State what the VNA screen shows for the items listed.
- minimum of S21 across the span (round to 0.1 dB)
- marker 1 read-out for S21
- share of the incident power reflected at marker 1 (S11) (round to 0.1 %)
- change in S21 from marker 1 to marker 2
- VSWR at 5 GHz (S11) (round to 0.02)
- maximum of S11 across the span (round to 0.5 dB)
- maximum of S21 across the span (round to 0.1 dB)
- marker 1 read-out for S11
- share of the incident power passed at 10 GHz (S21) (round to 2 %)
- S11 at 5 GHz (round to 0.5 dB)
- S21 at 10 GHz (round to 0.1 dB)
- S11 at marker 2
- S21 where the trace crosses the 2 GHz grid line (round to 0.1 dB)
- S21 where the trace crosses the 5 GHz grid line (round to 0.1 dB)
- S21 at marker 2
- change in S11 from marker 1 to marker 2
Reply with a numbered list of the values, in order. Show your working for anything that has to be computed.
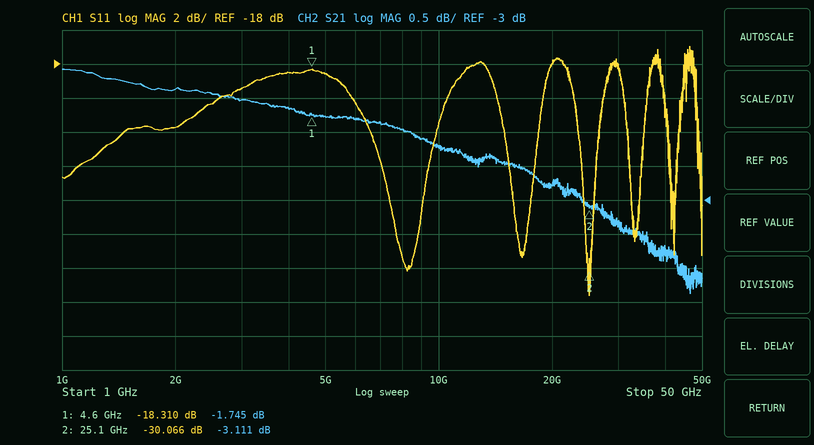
1. -4.4 dB
2. -1.745 dB
3. 10^(-18.31/10) ≈ 1.5 %
4. -3.111 − (-1.745) = -1.366 dB
5. |Γ| = 10^(-18.5/20) = 0.1189; VSWR = (1 + 0.1189)/(1 − 0.1189) ≈ 1.27, so 1.26 to the nearest 0.02
6. -17.0 dB
7. -1.1 dB
8. -18.310 dB
9. 10^(-2.2/10) ≈ 60 %
10. -18.5 dB
11. -2.2 dB
12. -30.066 dB
13. -1.4 dB
14. -1.8 dB
15. -3.111 dB
16. -30.066 − (-18.31) = -11.756 dB
